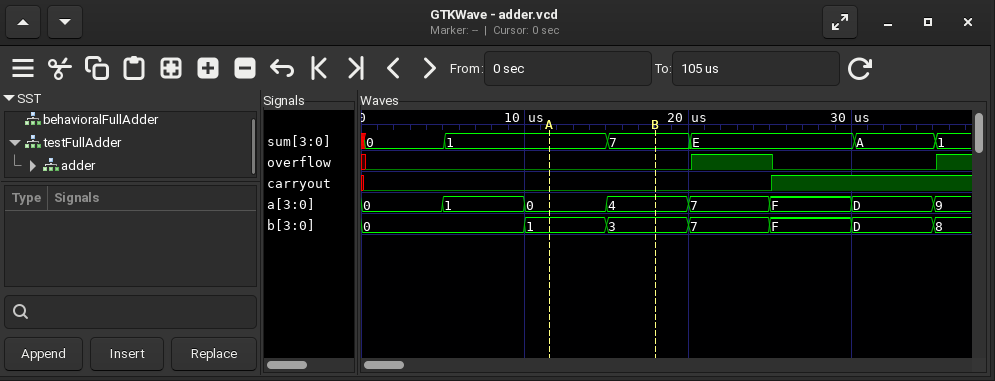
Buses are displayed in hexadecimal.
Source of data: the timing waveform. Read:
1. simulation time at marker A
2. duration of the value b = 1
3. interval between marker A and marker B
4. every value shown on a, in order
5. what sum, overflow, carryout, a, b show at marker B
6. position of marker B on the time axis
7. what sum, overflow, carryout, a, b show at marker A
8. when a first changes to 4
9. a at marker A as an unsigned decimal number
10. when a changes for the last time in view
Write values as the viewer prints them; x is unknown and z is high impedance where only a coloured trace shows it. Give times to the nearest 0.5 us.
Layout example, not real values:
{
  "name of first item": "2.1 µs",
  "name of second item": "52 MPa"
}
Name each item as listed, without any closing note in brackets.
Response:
{
  "simulation time at marker A": "11.5 us",
  "duration of the value b = 1": "5 us",
  "interval between marker A and marker B": "6.5 us",
  "every value shown on a, in order": "0, 1, 0, 4, 7, F, D, 9",
  "what sum, overflow, carryout, a, b show at marker B": "sum=7, overflow=0, carryout=0, a=4, b=3",
  "position of marker B on the time axis": "18 us",
  "what sum, overflow, carryout, a, b show at marker A": "sum=1, overflow=0, carryout=0, a=0, b=1",
  "when a first changes to 4": "15 us",
  "a at marker A as an unsigned decimal number": "0",
  "when a changes for the last time in view": "35 us"
}
